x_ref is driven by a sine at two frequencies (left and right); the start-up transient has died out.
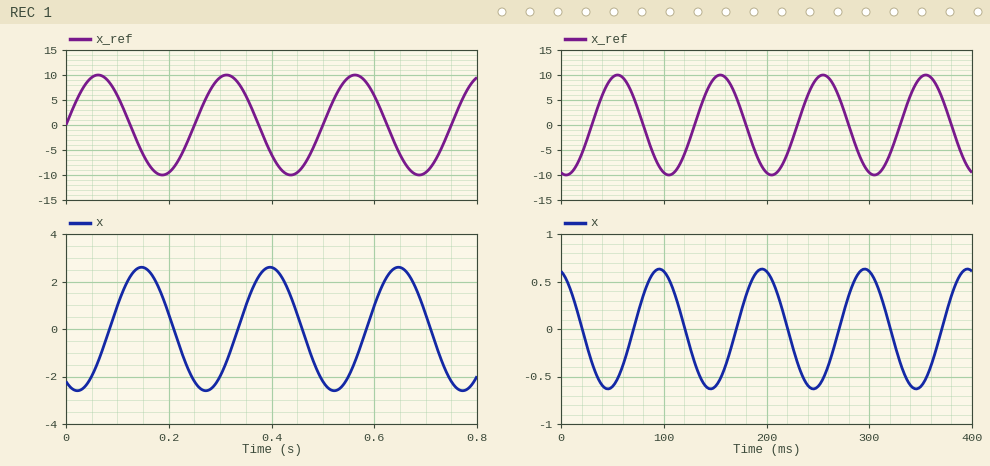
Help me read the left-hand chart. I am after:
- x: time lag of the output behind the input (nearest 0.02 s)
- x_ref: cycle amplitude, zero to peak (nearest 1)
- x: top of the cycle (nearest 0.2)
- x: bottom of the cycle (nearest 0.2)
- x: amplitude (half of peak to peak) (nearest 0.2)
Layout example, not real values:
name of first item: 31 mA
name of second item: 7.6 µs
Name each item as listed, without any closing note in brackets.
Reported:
x: time lag of the output behind the input: 0.08 s
x_ref: cycle amplitude, zero to peak: 10
x: top of the cycle: 2.6
x: bottom of the cycle: -2.6
x: amplitude (half of peak to peak): 2.6
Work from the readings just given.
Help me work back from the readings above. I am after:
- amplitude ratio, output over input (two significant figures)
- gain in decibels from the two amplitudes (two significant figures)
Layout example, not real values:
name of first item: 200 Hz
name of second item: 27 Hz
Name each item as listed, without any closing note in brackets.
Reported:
amplitude ratio, output over input: 0.26
gain in decibels from the two amplitudes: -12 dB
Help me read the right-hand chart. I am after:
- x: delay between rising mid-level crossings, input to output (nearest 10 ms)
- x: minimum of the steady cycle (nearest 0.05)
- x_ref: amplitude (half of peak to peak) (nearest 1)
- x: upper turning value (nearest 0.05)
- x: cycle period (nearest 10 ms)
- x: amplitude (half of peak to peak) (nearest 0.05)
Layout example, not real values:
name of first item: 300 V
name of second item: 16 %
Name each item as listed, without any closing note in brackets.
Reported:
x: delay between rising mid-level crossings, input to output: 40 ms
x: minimum of the steady cycle: -0.65
x_ref: amplitude (half of peak to peak): 10
x: upper turning value: 0.65
x: cycle period: 100 ms
x: amplitude (half of peak to peak): 0.65
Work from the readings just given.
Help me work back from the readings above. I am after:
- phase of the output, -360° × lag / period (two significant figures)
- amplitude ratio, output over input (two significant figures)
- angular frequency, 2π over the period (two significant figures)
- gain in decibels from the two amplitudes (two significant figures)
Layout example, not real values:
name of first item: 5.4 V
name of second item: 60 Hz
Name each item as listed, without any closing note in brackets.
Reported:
phase of the output, -360° × lag / period: -140°
amplitude ratio, output over input: 0.065
angular frequency, 2π over the period: 0.063 rad/ms
gain in decibels from the two amplitudes: -24 dB
